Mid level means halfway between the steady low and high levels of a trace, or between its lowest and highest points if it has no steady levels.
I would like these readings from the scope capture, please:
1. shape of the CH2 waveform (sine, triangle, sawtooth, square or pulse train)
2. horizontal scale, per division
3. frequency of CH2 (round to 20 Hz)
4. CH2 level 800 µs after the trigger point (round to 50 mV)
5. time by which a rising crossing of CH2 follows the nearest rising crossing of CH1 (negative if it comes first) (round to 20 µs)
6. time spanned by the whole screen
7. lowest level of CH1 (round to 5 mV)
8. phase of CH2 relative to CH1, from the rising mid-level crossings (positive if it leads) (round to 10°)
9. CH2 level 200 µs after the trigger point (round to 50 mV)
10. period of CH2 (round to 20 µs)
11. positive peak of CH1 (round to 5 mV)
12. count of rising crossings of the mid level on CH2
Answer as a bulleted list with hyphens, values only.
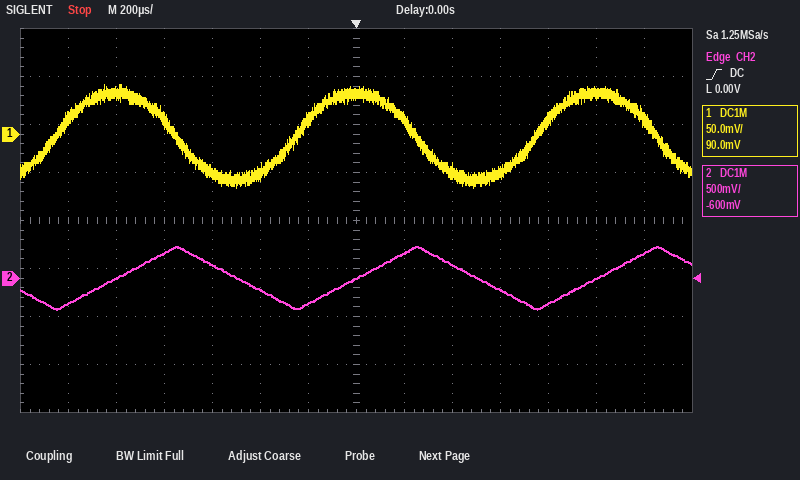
- triangle
- 200 µs
- 1.00 kHz
- -250 mV
- +260 µs
- 2.8 ms
- -55 mV
- -90°
- 250 mV
- 1.00 ms
- 50 mV
- 3
